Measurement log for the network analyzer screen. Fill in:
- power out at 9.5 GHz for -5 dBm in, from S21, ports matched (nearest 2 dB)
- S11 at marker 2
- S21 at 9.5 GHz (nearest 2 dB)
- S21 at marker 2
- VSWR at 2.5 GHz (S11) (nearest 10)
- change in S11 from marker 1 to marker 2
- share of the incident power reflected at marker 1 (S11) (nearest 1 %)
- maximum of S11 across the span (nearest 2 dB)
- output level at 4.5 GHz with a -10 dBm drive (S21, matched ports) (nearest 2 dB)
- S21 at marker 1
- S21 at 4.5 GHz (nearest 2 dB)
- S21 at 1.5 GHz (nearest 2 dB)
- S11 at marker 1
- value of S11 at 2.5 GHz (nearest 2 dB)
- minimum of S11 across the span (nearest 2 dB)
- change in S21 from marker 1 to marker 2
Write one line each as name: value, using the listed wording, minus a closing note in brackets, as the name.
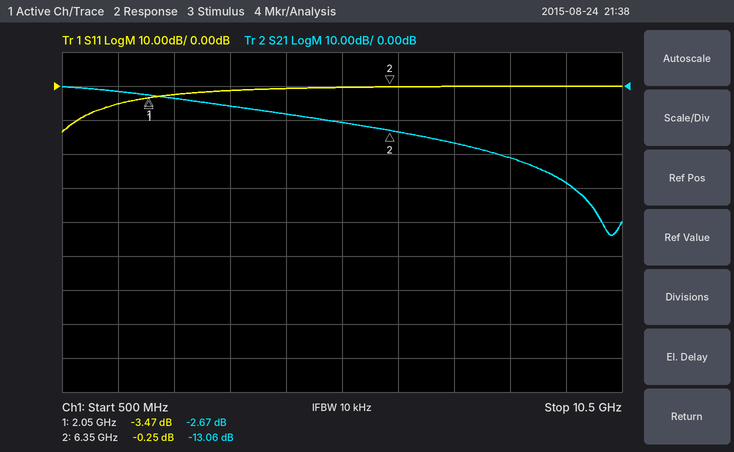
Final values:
power out at 9.5 GHz for -5 dBm in, from S21, ports matched: -34 dBm
S11 at marker 2: -0.25 dB
S21 at 9.5 GHz: -28 dB
S21 at marker 2: -13.06 dB
VSWR at 2.5 GHz (S11): 10
change in S11 from marker 1 to marker 2: 3.22 dB
share of the incident power reflected at marker 1 (S11): 45 %
maximum of S11 across the span: 0 dB
output level at 4.5 GHz with a -10 dBm drive (S21, matched ports): -18 dBm
S21 at marker 1: -2.67 dB
S21 at 4.5 GHz: -8 dB
S21 at 1.5 GHz: -2 dB
S11 at marker 1: -3.47 dB
value of S11 at 2.5 GHz: -2 dB
minimum of S11 across the span: -14 dB
change in S21 from marker 1 to marker 2: -10.39 dB
